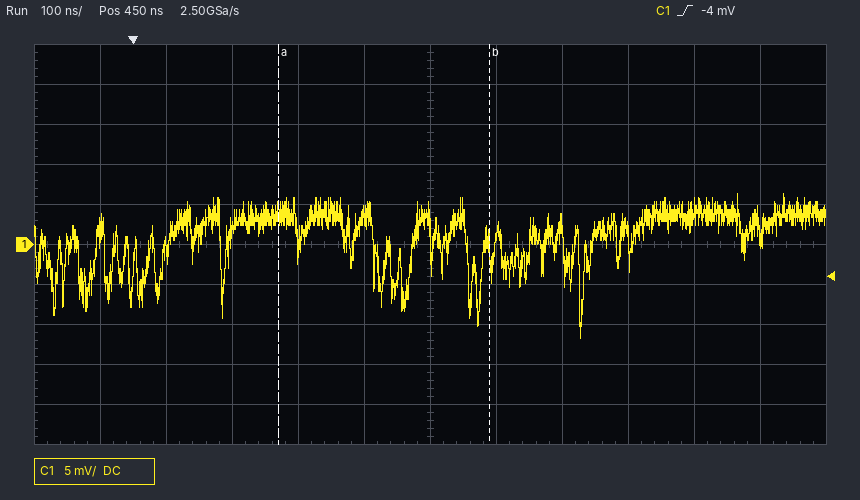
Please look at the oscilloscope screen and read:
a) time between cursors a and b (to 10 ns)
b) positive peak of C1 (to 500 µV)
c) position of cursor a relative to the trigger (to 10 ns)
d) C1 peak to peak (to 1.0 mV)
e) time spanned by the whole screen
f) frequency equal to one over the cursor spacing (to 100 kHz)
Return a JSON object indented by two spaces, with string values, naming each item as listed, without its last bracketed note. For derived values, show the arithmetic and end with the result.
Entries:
{
  "time between cursors a and b": "320 ns",
  "positive peak of C1": "6.5 mV",
  "position of cursor a relative to the trigger": "+220 ns",
  "C1 peak to peak": "18.0 mV",
  "time spanned by the whole screen": "1.2 µs",
  "frequency equal to one over the cursor spacing": "1 / 320 ns ≈ 3.1 MHz"
}
